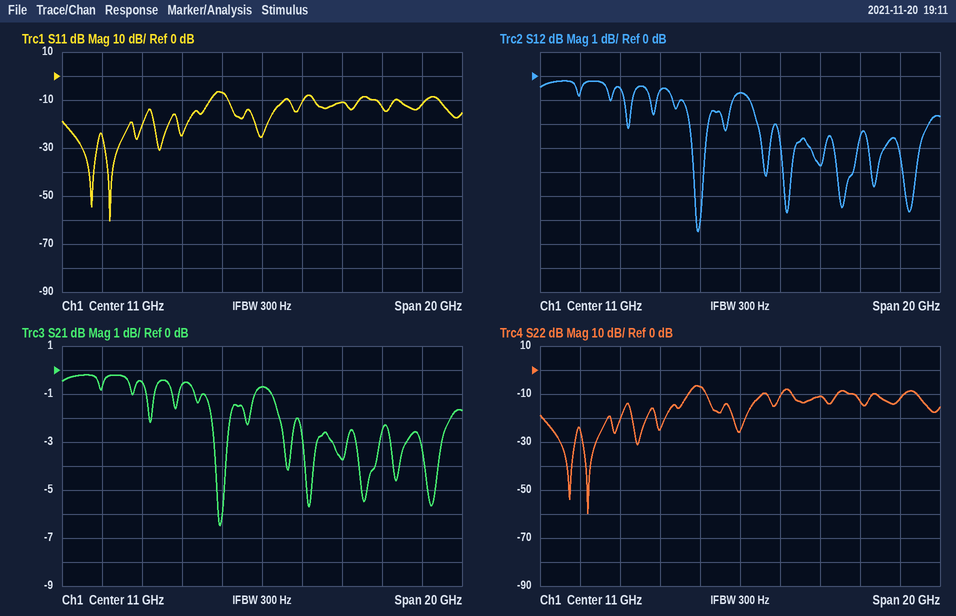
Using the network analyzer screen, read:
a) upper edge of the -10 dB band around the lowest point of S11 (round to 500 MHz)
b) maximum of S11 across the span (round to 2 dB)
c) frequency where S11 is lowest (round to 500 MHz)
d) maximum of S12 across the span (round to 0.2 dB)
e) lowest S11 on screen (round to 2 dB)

8.5 GHz
-6 dB
3.5 GHz
-0.2 dB
-60 dB
